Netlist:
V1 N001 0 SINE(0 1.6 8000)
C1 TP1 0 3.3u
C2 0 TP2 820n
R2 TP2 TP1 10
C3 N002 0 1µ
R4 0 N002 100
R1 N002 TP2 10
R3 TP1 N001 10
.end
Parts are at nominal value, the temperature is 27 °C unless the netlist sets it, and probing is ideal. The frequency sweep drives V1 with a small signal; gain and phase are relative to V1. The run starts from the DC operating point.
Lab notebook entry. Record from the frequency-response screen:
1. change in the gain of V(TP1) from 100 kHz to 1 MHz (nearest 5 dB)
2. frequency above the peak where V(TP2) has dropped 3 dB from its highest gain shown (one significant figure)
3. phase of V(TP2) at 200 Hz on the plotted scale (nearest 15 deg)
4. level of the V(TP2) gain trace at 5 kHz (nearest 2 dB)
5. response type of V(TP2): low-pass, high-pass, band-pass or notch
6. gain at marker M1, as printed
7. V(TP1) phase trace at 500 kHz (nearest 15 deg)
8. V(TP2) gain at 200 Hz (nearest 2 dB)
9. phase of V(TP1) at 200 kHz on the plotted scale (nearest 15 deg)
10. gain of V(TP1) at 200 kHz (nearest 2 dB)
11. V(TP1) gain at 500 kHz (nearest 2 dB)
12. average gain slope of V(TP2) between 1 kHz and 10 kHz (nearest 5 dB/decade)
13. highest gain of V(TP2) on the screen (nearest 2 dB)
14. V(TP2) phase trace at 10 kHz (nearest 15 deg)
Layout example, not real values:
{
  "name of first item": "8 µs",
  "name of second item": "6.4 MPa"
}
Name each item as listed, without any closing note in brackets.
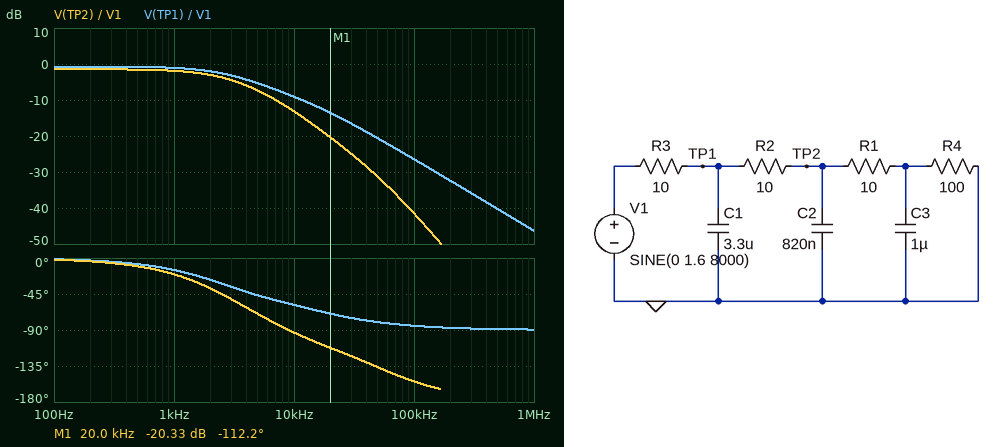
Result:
{
  "change in the gain of V(TP1) from 100 kHz to 1 MHz": "-20 dB",
  "frequency above the peak where V(TP2) has dropped 3 dB from its highest gain shown": "3 kHz",
  "phase of V(TP2) at 200 Hz on the plotted scale": "0 deg",
  "level of the V(TP2) gain trace at 5 kHz": "-8 dB",
  "response type of V(TP2): low-pass, high-pass, band-pass or notch": "low-pass",
  "gain at marker M1, as printed": "-20.33 dB",
  "V(TP1) phase trace at 500 kHz": "-90 deg",
  "V(TP2) gain at 200 Hz": "-2 dB",
  "phase of V(TP1) at 200 kHz on the plotted scale": "-90 deg",
  "gain of V(TP1) at 200 kHz": "-32 dB",
  "V(TP1) gain at 500 kHz": "-40 dB",
  "average gain slope of V(TP2) between 1 kHz and 10 kHz": "-10 dB/decade",
  "highest gain of V(TP2) on the screen": "-2 dB",
  "V(TP2) phase trace at 10 kHz": "-90 deg"
}
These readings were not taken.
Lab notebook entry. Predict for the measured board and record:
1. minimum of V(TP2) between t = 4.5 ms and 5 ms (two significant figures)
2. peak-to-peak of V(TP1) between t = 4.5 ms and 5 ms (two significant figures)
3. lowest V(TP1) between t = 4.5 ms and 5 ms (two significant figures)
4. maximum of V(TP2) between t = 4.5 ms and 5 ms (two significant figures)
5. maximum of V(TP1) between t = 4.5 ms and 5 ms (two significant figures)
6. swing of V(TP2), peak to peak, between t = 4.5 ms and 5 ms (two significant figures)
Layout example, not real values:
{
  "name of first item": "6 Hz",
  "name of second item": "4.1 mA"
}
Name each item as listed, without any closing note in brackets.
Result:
{
  "minimum of V(TP2) between t = 4.5 ms and 5 ms": "-450 mV",
  "peak-to-peak of V(TP1) between t = 4.5 ms and 5 ms": "1.3 V",
  "lowest V(TP1) between t = 4.5 ms and 5 ms": "-650 mV",
  "maximum of V(TP2) between t = 4.5 ms and 5 ms": "450 mV",
  "maximum of V(TP1) between t = 4.5 ms and 5 ms": "650 mV",
  "swing of V(TP2), peak to peak, between t = 4.5 ms and 5 ms": "890 mV"
}
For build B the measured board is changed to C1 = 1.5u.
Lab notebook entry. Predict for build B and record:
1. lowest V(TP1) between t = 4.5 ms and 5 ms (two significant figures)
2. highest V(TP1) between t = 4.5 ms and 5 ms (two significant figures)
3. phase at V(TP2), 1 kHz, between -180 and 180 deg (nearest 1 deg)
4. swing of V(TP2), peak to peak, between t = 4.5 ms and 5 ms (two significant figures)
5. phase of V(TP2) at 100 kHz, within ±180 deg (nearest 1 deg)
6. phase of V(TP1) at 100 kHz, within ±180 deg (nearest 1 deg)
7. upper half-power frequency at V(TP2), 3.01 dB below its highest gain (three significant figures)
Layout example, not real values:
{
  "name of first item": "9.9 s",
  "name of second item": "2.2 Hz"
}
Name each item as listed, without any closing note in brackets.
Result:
{
  "lowest V(TP1) between t = 4.5 ms and 5 ms": "-890 mV",
  "highest V(TP1) between t = 4.5 ms and 5 ms": "890 mV",
  "phase at V(TP2), 1 kHz, between -180 and 180 deg": "-15 deg",
  "swing of V(TP2), peak to peak, between t = 4.5 ms and 5 ms": "1.2 V",
  "phase of V(TP2) at 100 kHz, within ±180 deg": "-148 deg",
  "phase of V(TP1) at 100 kHz, within ±180 deg": "-79 deg",
  "upper half-power frequency at V(TP2), 3.01 dB below its highest gain": "4.02 kHz"
}
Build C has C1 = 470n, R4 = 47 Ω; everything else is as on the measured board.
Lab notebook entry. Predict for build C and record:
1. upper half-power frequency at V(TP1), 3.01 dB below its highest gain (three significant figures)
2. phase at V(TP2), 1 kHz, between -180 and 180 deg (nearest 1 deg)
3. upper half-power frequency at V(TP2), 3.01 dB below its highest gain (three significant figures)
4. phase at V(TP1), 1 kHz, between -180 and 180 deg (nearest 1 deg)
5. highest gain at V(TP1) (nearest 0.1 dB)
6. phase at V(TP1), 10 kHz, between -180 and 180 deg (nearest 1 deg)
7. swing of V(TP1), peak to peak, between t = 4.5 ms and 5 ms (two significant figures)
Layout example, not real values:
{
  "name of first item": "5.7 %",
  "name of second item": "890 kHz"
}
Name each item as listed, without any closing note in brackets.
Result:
{
  "upper half-power frequency at V(TP1), 3.01 dB below its highest gain": "10.7 kHz",
  "phase at V(TP2), 1 kHz, between -180 and 180 deg": "-9 deg",
  "upper half-power frequency at V(TP2), 3.01 dB below its highest gain": "5.97 kHz",
  "phase at V(TP1), 1 kHz, between -180 and 180 deg": "-5 deg",
  "highest gain at V(TP1)": "-1.2 dB",
  "phase at V(TP1), 10 kHz, between -180 and 180 deg": "-23 deg",
  "swing of V(TP1), peak to peak, between t = 4.5 ms and 5 ms": "2.1 V"
}
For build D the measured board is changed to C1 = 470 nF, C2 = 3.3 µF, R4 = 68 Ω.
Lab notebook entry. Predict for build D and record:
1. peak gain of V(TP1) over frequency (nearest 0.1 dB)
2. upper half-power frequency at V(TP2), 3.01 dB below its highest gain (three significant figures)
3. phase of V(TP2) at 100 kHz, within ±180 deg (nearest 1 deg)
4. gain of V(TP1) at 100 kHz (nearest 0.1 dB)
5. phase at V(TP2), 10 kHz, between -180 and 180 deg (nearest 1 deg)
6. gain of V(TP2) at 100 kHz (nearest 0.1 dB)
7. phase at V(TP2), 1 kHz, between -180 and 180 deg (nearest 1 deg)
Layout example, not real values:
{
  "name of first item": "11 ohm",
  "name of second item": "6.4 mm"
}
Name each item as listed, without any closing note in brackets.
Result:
{
  "peak gain of V(TP1) over frequency": "-0.9 dB",
  "upper half-power frequency at V(TP2), 3.01 dB below its highest gain": "2.34 kHz",
  "phase of V(TP2) at 100 kHz, within ±180 deg": "-141 deg",
  "gain of V(TP1) at 100 kHz": "-11.1 dB",
  "phase at V(TP2), 10 kHz, between -180 and 180 deg": "-80 deg",
  "gain of V(TP2) at 100 kHz": "-37.6 dB",
  "phase at V(TP2), 1 kHz, between -180 and 180 deg": "-23 deg"
}
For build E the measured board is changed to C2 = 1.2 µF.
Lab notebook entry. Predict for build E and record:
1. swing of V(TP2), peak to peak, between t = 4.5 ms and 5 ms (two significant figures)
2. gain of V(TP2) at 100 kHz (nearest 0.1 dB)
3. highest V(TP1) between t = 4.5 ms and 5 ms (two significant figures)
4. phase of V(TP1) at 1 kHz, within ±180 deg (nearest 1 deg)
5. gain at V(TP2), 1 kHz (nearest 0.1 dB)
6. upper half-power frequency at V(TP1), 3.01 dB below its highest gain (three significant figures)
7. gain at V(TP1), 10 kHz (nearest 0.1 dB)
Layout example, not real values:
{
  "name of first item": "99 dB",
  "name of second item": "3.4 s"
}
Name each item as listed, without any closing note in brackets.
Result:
{
  "swing of V(TP2), peak to peak, between t = 4.5 ms and 5 ms": "810 mV",
  "gain of V(TP2) at 100 kHz": "-44.4 dB",
  "highest V(TP1) between t = 4.5 ms and 5 ms": "630 mV",
  "phase of V(TP1) at 1 kHz, within ±180 deg": "-16 deg",
  "gain at V(TP2), 1 kHz": "-2.0 dB",
  "upper half-power frequency at V(TP1), 3.01 dB below its highest gain": "3.18 kHz",
  "gain at V(TP1), 10 kHz": "-9.3 dB"
}
